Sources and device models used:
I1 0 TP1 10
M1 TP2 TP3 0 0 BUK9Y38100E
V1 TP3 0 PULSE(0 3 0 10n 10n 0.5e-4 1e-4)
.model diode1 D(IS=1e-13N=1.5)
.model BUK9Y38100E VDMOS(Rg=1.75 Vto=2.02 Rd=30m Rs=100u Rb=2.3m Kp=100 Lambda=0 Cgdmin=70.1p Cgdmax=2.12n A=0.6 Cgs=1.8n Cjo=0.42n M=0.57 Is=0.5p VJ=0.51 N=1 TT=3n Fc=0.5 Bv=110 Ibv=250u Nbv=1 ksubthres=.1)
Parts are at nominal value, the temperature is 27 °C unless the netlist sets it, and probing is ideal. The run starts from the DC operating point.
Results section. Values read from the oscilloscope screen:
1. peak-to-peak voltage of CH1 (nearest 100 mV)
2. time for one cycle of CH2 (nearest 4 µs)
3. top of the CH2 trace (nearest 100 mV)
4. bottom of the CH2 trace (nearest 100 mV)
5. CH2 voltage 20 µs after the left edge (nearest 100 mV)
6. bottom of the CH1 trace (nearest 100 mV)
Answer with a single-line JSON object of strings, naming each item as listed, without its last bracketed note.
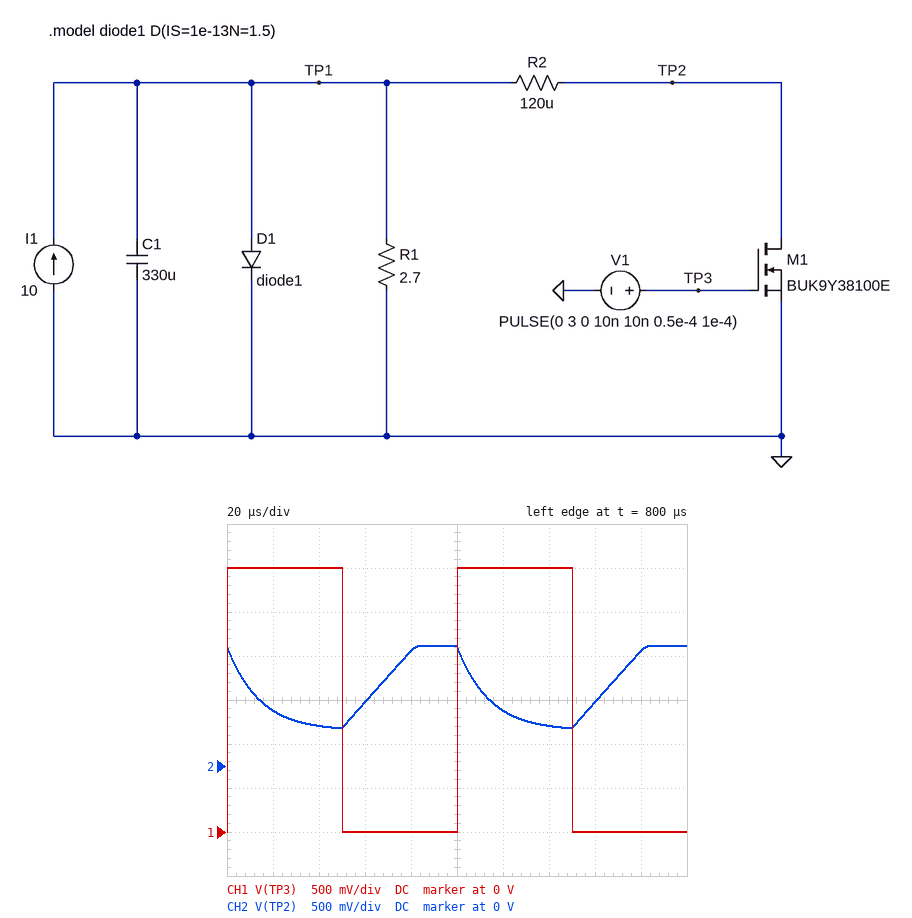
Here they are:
{"peak-to-peak voltage of CH1": "3.0 V", "time for one cycle of CH2": "100 µs", "top of the CH2 trace": "1.4 V", "bottom of the CH2 trace": "400 mV", "CH2 voltage 20 µs after the left edge": "600 mV", "bottom of the CH1 trace": "0 V"}
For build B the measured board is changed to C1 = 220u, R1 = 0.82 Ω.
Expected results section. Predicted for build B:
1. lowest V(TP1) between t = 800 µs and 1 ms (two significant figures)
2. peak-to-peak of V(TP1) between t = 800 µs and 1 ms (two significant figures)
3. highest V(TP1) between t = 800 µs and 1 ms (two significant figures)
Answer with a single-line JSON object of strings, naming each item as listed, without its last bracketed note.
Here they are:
{"lowest V(TP1) between t = 800 µs and 1 ms": "390 mV", "peak-to-peak of V(TP1) between t = 800 µs and 1 ms": "970 mV", "highest V(TP1) between t = 800 µs and 1 ms": "1.4 V"}
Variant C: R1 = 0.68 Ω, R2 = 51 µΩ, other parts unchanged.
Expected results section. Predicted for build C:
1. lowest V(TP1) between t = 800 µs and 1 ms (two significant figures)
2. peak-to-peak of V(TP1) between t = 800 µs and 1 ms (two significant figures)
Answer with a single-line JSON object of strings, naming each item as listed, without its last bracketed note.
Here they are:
{"lowest V(TP1) between t = 800 µs and 1 ms": "410 mV", "peak-to-peak of V(TP1) between t = 800 µs and 1 ms": "960 mV"}
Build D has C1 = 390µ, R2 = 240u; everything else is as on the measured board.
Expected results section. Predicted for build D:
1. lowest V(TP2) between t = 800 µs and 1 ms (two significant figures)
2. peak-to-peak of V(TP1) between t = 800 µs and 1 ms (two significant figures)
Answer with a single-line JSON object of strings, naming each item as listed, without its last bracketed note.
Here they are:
{"lowest V(TP2) between t = 800 µs and 1 ms": "450 mV", "peak-to-peak of V(TP1) between t = 800 µs and 1 ms": "920 mV"}
